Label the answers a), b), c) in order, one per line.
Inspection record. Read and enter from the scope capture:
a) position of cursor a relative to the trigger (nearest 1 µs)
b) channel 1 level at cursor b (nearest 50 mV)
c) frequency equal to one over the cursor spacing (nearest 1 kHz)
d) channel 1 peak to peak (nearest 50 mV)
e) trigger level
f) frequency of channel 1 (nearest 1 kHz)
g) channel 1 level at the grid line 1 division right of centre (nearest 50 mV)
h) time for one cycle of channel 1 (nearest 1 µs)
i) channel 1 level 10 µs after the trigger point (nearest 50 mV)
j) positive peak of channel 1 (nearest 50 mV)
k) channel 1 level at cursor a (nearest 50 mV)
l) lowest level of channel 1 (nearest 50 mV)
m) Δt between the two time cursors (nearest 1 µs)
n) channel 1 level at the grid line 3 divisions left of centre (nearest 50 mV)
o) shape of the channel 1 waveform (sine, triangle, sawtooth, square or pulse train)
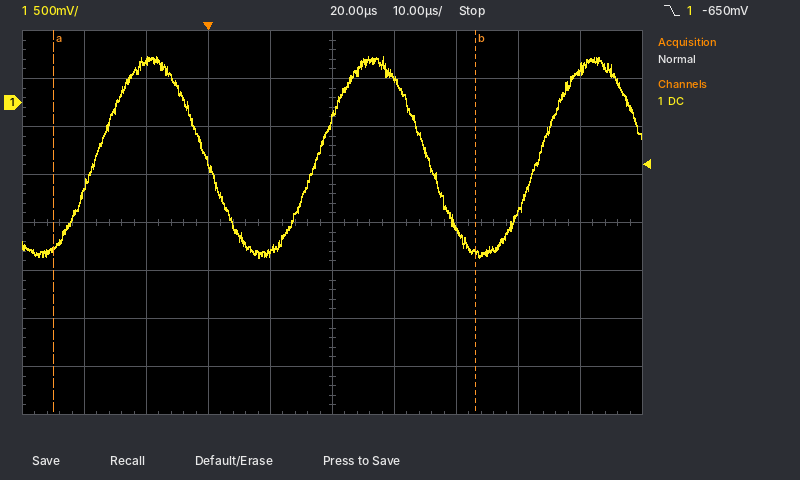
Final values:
a) -25 µs
b) -1.55 V
c) 15 kHz
d) 2.10 V
e) -650 mV
f) 28 kHz
g) 250 mV
h) 36 µs
i) -1.55 V
j) 500 mV
k) -1.50 V
l) -1.60 V
m) 68 µs
n) 450 mV
o) sine
